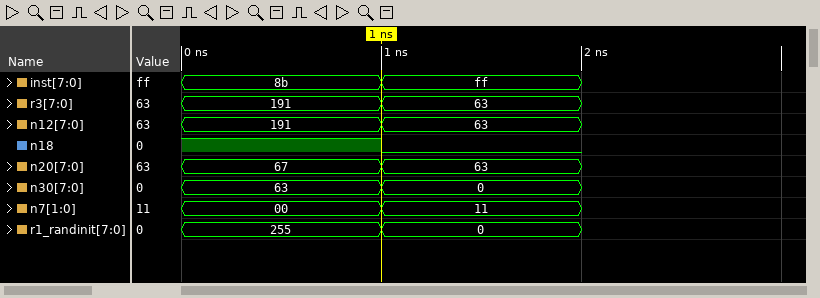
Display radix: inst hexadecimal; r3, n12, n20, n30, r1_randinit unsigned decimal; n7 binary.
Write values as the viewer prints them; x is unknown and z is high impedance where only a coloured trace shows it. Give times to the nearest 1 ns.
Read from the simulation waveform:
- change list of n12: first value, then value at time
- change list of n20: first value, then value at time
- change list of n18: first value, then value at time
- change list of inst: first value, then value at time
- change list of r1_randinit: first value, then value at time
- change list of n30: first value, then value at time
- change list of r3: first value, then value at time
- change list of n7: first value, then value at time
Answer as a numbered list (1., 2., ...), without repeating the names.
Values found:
1. 191, 63 at 1 ns
2. 67, 63 at 1 ns
3. 1, 0 at 1 ns
4. 8b, ff at 1 ns
5. 255, 0 at 1 ns
6. 63, 0 at 1 ns
7. 191, 63 at 1 ns
8. 00, 11 at 1 ns
